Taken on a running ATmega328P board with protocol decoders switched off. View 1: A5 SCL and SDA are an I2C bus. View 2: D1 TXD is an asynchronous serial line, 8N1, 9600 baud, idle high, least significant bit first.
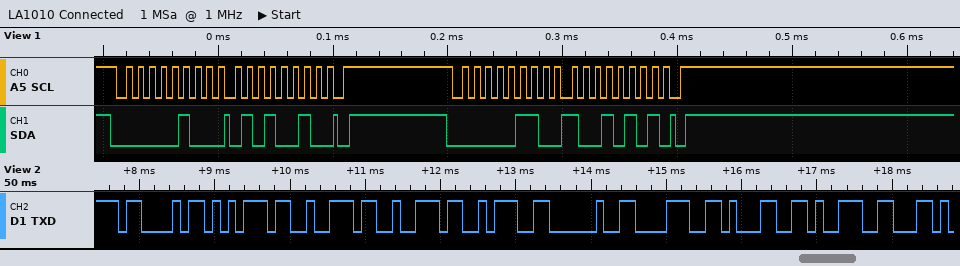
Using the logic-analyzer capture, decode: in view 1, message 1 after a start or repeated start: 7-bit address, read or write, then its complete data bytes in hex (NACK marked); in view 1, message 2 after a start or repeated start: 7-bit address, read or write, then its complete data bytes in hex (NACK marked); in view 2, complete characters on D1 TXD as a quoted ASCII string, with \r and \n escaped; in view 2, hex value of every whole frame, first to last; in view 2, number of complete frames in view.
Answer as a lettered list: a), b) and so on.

a) 0x02 write: 52
b) 0x03 write: 95
c) "Curr: 819"
d) 43 75 72 72 3A 20 38 31 39
e) 9
